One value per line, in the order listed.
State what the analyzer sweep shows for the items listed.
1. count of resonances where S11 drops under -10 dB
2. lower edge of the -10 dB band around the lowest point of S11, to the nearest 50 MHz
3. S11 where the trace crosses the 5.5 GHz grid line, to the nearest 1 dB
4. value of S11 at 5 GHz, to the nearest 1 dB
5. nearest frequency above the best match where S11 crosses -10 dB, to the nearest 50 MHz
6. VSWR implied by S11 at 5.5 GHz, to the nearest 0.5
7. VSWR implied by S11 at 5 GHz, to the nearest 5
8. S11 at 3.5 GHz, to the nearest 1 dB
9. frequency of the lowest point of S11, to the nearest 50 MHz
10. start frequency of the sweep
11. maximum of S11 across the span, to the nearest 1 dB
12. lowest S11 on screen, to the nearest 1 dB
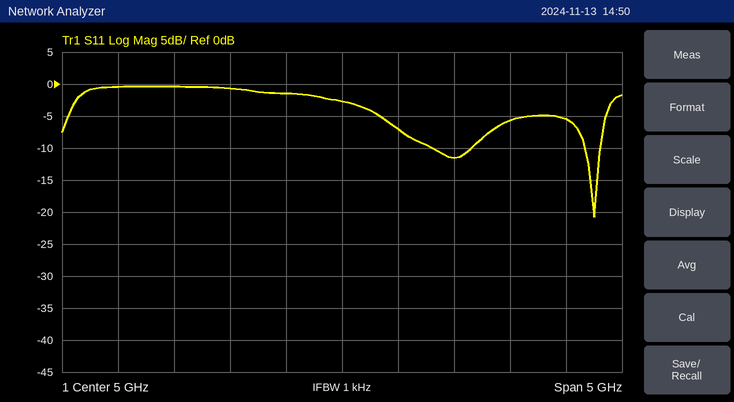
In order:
2
7.15 GHz
-7 dB
-3 dB
7.30 GHz
2.5
5
0 dB
7.25 GHz
2.5 GHz
0 dB
-21 dB
